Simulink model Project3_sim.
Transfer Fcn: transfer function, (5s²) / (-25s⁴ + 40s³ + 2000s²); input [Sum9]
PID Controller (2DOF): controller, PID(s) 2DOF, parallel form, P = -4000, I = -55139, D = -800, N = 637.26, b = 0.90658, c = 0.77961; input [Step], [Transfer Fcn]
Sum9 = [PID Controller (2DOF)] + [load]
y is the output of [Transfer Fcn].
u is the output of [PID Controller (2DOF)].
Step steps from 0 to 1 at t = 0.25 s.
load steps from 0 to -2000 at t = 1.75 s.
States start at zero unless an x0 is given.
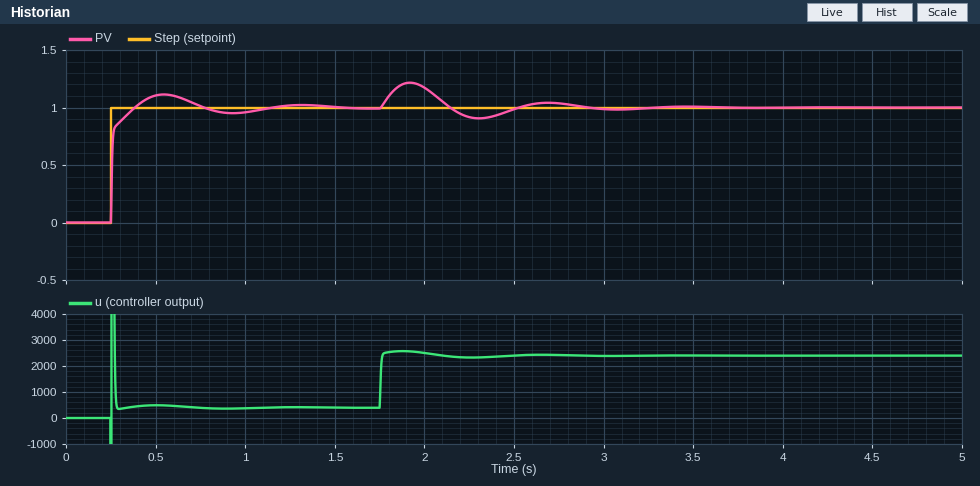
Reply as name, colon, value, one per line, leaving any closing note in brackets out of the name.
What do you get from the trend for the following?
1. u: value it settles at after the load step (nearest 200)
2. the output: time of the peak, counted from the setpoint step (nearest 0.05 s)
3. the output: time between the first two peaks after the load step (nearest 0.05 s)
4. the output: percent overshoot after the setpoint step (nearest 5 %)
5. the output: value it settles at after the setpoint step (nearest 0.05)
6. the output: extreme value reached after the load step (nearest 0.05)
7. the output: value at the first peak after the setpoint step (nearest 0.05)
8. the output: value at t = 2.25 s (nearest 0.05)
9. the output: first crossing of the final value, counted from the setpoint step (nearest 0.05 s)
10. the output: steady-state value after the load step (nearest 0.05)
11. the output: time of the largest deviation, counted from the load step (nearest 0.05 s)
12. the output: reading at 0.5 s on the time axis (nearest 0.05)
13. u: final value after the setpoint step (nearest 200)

u: value it settles at after the load step: 2400
the output: time of the peak, counted from the setpoint step: 0.30 s
the output: time between the first two peaks after the load step: 0.75 s
the output: percent overshoot after the setpoint step: 10 %
the output: value it settles at after the setpoint step: 1.00
the output: extreme value reached after the load step: 1.20
the output: value at the first peak after the setpoint step: 1.10
the output: value at t = 2.25 s: 0.90
the output: first crossing of the final value, counted from the setpoint step: 0.15 s
the output: steady-state value after the load step: 1.00
the output: time of the largest deviation, counted from the load step: 0.15 s
the output: reading at 0.5 s on the time axis: 1.10
u: final value after the setpoint step: 400
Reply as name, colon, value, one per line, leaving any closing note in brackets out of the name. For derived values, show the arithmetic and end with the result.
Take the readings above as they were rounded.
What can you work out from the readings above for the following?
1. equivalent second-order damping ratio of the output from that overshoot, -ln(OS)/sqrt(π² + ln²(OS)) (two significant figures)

equivalent second-order damping ratio of the output from that overshoot, -ln(OS)/sqrt(π² + ln²(OS)): ln(0.1) = -2.303; 2.303 / sqrt(9.870 + 5.302) = 0.59
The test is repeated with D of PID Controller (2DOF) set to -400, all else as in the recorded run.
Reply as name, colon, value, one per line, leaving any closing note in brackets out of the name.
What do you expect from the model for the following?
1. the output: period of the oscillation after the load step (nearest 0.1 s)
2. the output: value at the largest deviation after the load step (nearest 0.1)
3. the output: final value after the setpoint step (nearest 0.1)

the output: period of the oscillation after the load step: 0.5 s
the output: value at the largest deviation after the load step: 1.3
the output: final value after the setpoint step: 1.0
